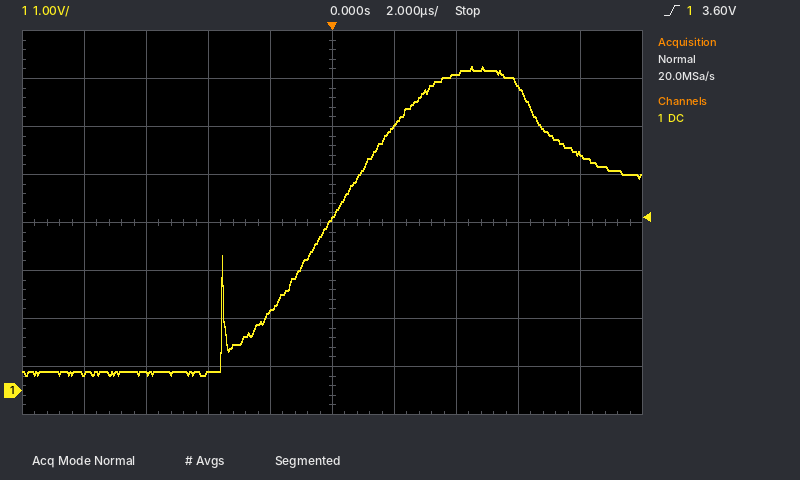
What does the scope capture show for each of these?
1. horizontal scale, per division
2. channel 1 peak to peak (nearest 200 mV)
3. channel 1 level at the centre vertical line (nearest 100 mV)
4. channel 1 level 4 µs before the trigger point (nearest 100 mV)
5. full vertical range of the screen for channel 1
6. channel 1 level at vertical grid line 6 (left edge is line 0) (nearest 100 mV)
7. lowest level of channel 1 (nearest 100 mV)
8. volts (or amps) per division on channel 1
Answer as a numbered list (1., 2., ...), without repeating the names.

1. 2 µs
2. 6.4 V
3. 3.6 V
4. 400 mV
5. 8 V
6. 5.5 V
7. 300 mV
8. 1 V
